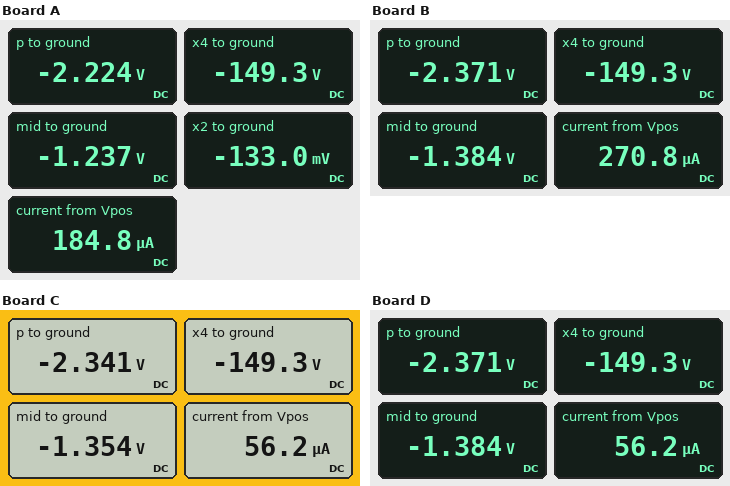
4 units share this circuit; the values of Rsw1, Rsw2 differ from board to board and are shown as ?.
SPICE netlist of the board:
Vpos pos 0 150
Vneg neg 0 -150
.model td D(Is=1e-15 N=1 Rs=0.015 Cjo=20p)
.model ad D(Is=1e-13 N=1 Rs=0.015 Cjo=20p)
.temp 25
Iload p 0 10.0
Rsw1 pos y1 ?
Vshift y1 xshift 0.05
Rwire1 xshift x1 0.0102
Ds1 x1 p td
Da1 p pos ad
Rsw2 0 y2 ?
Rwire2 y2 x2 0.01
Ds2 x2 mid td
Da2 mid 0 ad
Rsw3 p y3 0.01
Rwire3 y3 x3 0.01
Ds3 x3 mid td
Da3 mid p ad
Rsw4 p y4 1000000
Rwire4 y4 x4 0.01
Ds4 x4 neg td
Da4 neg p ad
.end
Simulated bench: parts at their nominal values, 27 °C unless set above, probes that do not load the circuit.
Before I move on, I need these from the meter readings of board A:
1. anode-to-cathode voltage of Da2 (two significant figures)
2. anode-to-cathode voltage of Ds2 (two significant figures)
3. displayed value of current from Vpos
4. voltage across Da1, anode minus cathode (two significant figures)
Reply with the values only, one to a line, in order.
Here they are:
-1.2 V
1.1 V
184.8 µA
-150 V
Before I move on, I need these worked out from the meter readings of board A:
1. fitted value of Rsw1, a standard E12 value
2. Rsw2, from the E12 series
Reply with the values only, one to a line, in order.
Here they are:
820 kΩ
3.3 mΩ
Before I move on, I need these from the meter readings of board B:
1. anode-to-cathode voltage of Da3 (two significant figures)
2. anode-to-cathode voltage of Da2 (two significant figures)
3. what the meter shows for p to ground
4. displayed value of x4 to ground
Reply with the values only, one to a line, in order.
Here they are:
990 mV
-1.4 V
-2.371 V
-149.3 V
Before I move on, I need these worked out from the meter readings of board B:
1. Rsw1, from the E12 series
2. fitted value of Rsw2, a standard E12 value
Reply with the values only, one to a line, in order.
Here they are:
560 kΩ
0.018 Ω
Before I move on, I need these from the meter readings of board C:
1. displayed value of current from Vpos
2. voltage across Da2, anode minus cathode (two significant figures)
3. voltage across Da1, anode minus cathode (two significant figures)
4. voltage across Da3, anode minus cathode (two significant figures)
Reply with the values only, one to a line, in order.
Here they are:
56.2 µA
-1.4 V
-150 V
990 mV
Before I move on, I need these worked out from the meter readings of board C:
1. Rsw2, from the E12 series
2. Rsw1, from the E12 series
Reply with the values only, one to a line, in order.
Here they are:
0.015 Ω
2.7 MΩ
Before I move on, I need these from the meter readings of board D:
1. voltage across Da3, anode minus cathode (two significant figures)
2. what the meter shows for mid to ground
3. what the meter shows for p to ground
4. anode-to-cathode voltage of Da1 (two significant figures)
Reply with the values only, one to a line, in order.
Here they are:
990 mV
-1.384 V
-2.371 V
-150 V
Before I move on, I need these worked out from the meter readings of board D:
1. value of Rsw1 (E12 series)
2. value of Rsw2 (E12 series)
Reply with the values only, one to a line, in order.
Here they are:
2.7 MΩ
0.018 Ω
